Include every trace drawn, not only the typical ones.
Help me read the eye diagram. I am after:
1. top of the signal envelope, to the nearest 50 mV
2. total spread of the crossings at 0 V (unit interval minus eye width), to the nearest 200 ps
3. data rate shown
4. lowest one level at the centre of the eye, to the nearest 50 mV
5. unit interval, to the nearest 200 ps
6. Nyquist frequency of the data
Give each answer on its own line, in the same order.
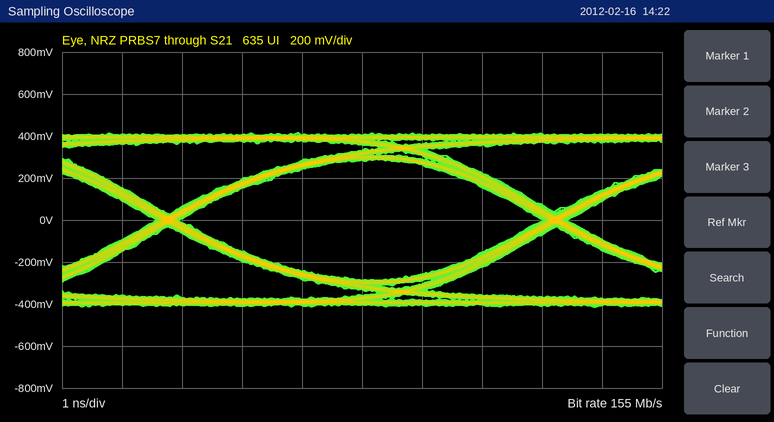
400 mV
400 ps
155 Mb/s
300 mV
6.4 ns
77.5 MHz
